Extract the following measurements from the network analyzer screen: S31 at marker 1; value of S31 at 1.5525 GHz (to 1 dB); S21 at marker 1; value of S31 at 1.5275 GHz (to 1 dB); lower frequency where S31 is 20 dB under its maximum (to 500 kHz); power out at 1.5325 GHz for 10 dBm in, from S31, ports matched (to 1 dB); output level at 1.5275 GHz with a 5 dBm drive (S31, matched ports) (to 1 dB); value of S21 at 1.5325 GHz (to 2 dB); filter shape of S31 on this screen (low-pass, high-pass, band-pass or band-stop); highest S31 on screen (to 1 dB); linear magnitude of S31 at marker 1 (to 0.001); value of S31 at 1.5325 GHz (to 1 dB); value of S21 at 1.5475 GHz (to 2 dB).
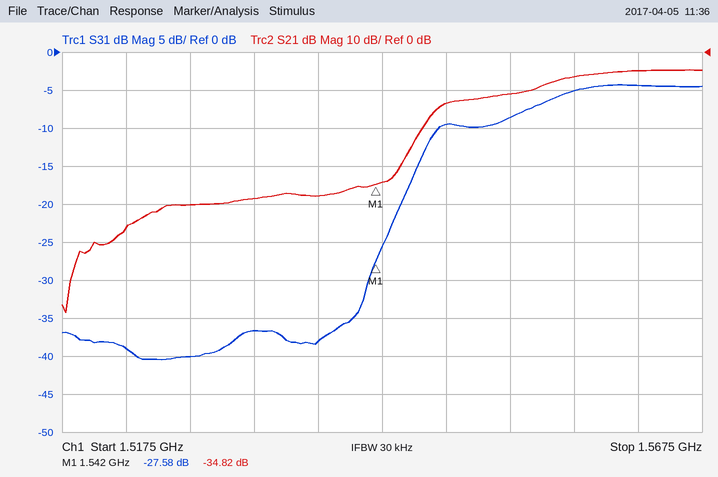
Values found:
-27.58 dB
-9 dB
-34.82 dB
-40 dB
1.5430 GHz
-27 dBm
-35 dBm
-38 dB
high-pass
-4 dB
0.042
-37 dB
-14 dB
